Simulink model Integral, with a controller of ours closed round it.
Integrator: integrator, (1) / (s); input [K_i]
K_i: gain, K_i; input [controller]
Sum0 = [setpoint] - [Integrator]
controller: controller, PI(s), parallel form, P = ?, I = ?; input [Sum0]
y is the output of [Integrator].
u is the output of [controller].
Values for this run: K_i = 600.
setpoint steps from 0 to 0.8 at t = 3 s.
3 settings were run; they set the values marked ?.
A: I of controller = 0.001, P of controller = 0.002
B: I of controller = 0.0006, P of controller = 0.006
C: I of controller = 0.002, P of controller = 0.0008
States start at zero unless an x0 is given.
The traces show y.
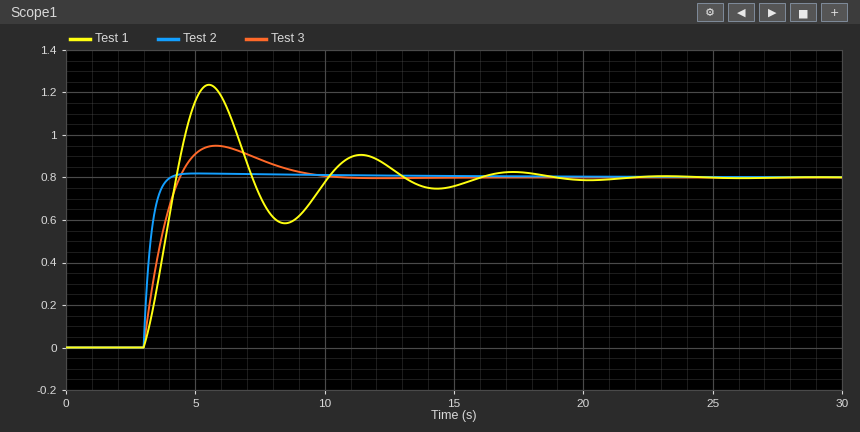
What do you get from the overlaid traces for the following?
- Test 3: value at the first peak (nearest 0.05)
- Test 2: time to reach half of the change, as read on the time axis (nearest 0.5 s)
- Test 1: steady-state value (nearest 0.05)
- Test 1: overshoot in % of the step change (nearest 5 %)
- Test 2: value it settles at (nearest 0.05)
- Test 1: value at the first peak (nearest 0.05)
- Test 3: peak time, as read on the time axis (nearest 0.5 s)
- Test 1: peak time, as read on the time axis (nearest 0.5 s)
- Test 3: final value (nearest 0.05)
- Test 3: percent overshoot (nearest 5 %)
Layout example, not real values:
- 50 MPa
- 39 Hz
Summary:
- 0.95
- 3.0 s
- 0.80
- 55 %
- 0.80
- 1.25
- 6.0 s
- 5.5 s
- 0.80
- 20 %
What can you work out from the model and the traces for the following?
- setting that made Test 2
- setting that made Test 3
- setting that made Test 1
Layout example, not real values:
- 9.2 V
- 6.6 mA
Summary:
- B
- A
- C
